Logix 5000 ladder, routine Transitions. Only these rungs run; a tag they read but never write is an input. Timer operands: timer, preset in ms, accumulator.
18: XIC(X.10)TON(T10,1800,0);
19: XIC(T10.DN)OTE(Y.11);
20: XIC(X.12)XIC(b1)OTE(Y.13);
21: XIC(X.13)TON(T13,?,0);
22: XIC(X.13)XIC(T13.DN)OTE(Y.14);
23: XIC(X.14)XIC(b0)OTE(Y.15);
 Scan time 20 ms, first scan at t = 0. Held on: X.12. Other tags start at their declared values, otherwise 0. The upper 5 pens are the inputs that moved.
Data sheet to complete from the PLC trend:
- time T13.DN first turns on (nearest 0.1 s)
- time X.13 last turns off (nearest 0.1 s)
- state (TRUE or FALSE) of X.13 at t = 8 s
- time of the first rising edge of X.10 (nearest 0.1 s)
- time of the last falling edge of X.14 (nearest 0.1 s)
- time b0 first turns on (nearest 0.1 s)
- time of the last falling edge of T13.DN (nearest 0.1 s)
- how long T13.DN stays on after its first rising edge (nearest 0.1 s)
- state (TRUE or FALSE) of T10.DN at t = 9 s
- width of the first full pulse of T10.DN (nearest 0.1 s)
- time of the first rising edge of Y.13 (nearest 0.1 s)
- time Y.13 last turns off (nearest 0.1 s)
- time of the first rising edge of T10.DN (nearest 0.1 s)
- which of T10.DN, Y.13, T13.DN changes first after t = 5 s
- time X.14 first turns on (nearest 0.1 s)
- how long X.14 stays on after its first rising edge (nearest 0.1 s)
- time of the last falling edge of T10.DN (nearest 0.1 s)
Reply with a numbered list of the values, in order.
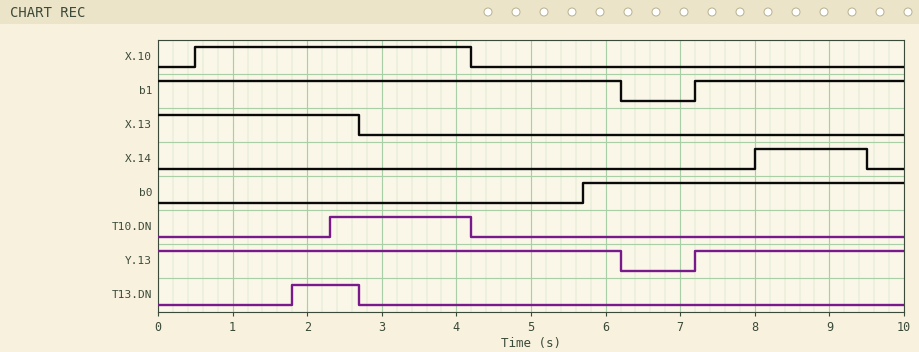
1. 1.8 s
2. 2.7 s
3. FALSE
4. 0.5 s
5. 9.5 s
6. 5.7 s
7. 2.7 s
8. 0.9 s
9. FALSE
10. 1.9 s
11. 7.2 s
12. 6.2 s
13. 2.3 s
14. Y.13
15. 8.0 s
16. 1.5 s
17. 4.2 s
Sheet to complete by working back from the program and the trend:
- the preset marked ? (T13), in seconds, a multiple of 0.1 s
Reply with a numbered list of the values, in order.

1. 1.8 s
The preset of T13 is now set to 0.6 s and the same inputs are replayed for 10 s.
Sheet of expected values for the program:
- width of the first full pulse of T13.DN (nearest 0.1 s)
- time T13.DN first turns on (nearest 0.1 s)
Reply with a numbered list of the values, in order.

1. 2.1 s
2. 0.6 s
